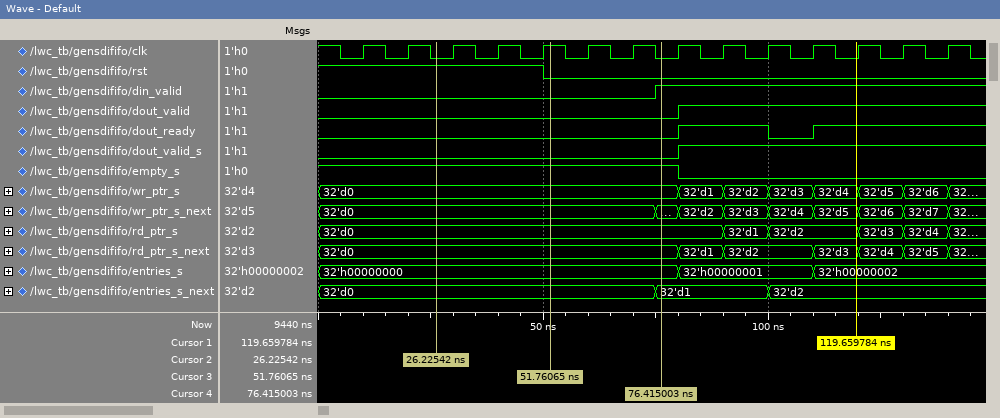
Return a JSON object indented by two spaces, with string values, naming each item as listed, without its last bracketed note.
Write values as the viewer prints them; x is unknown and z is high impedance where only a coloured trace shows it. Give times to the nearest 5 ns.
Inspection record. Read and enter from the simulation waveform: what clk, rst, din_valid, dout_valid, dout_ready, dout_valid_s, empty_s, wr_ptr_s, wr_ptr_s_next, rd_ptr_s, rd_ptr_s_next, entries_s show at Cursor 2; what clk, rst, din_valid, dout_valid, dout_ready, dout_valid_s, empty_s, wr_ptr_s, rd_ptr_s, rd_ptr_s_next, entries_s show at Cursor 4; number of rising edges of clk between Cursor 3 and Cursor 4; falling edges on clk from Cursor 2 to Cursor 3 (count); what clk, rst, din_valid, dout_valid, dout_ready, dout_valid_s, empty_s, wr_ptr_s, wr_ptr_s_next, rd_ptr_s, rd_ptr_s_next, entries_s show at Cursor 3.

{
  "what clk, rst, din_valid, dout_valid, dout_ready, dout_valid_s, empty_s, wr_ptr_s, wr_ptr_s_next, rd_ptr_s, rd_ptr_s_next, entries_s show at Cursor 2": "clk=0, rst=1, din_valid=0, dout_valid=0, dout_ready=0, dout_valid_s=0, empty_s=1, wr_ptr_s=32'd0, wr_ptr_s_next=32'd0, rd_ptr_s=32'd0, rd_ptr_s_next=32'd0, entries_s=32'h00000000",
  "what clk, rst, din_valid, dout_valid, dout_ready, dout_valid_s, empty_s, wr_ptr_s, rd_ptr_s, rd_ptr_s_next, entries_s show at Cursor 4": "clk=0, rst=0, din_valid=1, dout_valid=0, dout_ready=0, dout_valid_s=0, empty_s=1, wr_ptr_s=32'd0, rd_ptr_s=32'd0, rd_ptr_s_next=32'd0, entries_s=32'h00000000",
  "number of rising edges of clk between Cursor 3 and Cursor 4": "2",
  "falling edges on clk from Cursor 2 to Cursor 3": "2",
  "what clk, rst, din_valid, dout_valid, dout_ready, dout_valid_s, empty_s, wr_ptr_s, wr_ptr_s_next, rd_ptr_s, rd_ptr_s_next, entries_s show at Cursor 3": "clk=1, rst=0, din_valid=0, dout_valid=0, dout_ready=0, dout_valid_s=0, empty_s=1, wr_ptr_s=32'd0, wr_ptr_s_next=32'd0, rd_ptr_s=32'd0, rd_ptr_s_next=32'd0, entries_s=32'h00000000"
}
